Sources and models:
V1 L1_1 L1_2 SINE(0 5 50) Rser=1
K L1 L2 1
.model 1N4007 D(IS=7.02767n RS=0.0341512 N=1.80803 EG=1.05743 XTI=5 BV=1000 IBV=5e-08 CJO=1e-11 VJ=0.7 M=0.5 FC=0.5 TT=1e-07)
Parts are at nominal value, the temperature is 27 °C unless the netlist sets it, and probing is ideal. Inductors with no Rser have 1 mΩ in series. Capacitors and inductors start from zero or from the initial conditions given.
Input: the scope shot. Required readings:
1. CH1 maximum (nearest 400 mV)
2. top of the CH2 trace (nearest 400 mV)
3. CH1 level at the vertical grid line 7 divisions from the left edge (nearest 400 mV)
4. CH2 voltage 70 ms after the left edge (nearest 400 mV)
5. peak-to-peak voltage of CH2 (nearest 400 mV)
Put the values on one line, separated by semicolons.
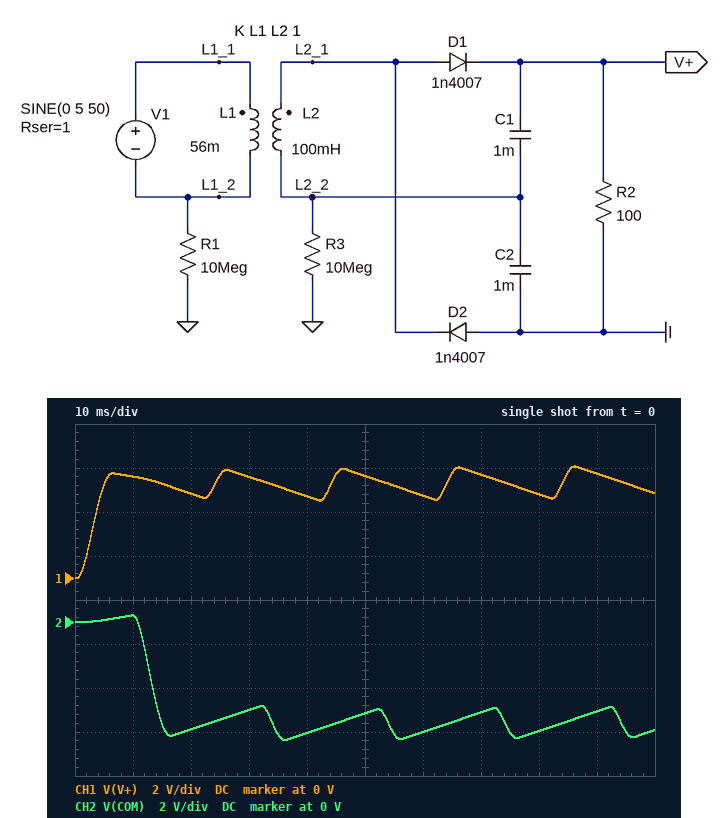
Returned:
5.2 V; 400 mV; 4.8 V; -4.0 V; 5.6 V
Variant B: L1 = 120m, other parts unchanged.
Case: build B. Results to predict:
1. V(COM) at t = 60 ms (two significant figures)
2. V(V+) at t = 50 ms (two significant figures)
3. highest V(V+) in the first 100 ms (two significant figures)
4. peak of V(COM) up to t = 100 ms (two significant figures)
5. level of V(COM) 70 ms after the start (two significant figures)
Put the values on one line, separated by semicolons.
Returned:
-3.4 V; 3.2 V; 3.5 V; 240 mV; -2.8 V
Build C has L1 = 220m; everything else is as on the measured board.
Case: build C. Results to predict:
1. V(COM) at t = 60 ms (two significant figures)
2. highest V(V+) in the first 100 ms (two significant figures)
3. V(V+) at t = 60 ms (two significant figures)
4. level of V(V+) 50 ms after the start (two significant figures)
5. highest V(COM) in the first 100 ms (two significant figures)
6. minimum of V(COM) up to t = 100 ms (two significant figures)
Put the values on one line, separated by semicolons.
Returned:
-2.4 V; 2.5 V; 1.9 V; 2.3 V; 180 mV; -2.6 V
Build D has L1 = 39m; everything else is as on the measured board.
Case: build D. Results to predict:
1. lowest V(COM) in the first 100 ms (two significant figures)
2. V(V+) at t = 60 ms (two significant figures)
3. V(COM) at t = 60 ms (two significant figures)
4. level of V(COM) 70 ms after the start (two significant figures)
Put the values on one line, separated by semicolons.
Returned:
-6.3 V; 4.3 V; -5.8 V; -4.8 V
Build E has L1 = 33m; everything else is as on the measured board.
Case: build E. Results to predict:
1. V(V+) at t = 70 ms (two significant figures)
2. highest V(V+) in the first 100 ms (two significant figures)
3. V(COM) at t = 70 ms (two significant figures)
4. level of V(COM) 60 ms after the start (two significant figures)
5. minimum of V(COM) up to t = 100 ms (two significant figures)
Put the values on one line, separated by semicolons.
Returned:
5.8 V; 6.3 V; -5.1 V; -6.2 V; -6.7 V
